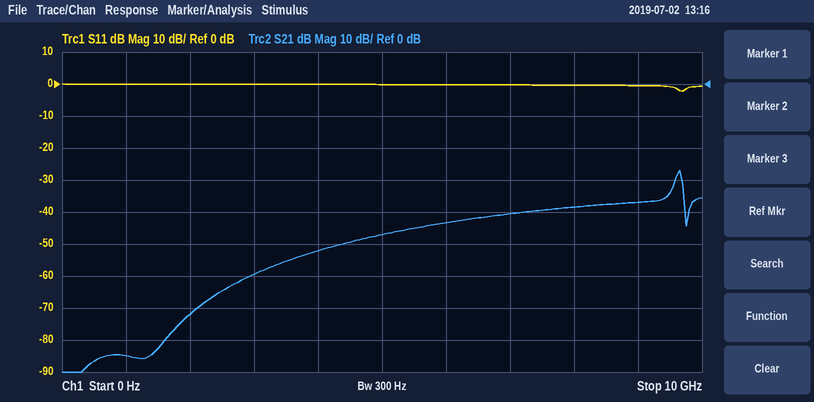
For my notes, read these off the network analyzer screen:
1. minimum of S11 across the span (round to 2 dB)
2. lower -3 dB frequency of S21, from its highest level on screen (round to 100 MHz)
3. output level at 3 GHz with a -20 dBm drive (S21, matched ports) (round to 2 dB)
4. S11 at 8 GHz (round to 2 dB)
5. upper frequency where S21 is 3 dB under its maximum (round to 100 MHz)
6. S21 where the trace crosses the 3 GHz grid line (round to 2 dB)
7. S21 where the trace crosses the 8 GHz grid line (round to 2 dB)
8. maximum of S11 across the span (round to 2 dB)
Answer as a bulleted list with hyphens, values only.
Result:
- -2 dB
- 9.6 GHz
- -80 dBm
- 0 dB
- 9.7 GHz
- -60 dB
- -38 dB
- 0 dB
